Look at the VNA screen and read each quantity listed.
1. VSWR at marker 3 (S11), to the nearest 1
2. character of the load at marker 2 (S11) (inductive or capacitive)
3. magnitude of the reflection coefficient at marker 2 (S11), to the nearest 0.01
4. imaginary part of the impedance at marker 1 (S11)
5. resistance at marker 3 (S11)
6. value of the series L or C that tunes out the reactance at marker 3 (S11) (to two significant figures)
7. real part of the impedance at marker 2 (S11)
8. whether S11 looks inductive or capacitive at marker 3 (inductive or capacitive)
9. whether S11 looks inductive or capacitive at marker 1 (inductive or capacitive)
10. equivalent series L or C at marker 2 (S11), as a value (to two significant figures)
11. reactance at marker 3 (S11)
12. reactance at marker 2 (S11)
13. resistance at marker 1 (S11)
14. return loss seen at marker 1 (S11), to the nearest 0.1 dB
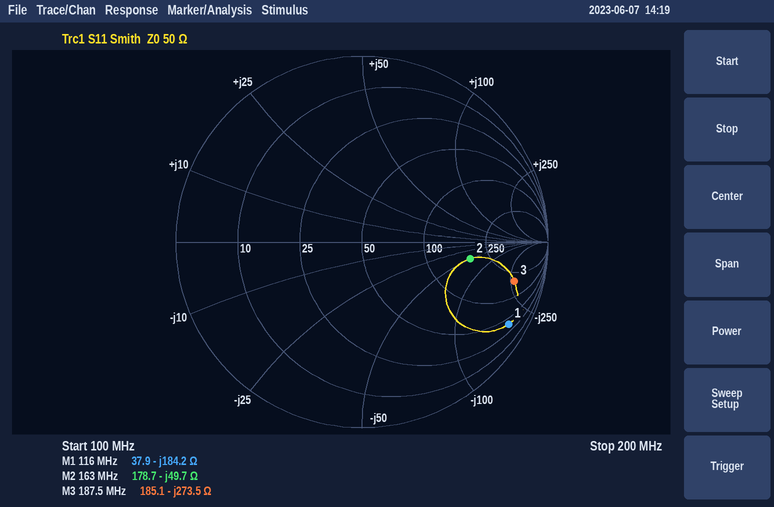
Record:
12
capacitive
0.59
-184.2 Ω
185.1 Ω
230 nH
178.7 Ω
capacitive
capacitive
20 pF
-273.5 Ω
-49.7 Ω
37.9 Ω
0.9 dB
